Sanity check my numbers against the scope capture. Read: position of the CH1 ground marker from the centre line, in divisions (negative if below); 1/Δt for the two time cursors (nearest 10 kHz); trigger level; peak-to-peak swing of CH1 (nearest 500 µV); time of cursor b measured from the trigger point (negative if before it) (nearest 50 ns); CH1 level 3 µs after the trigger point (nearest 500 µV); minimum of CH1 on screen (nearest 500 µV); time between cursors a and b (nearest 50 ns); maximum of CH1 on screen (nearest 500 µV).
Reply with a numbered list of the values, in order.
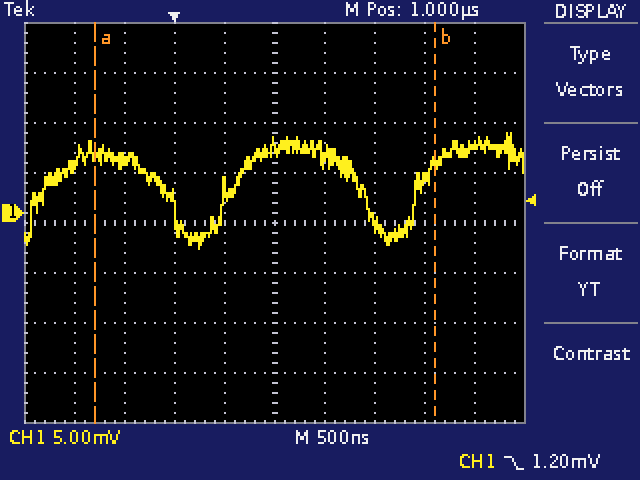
1. +0.2 div
2. 290 kHz
3. 1.20 mV
4. 11.5 mV
5. +2.60 µs
6. 7.0 mV
7. -3.5 mV
8. 3.40 µs
9. 8.0 mV
